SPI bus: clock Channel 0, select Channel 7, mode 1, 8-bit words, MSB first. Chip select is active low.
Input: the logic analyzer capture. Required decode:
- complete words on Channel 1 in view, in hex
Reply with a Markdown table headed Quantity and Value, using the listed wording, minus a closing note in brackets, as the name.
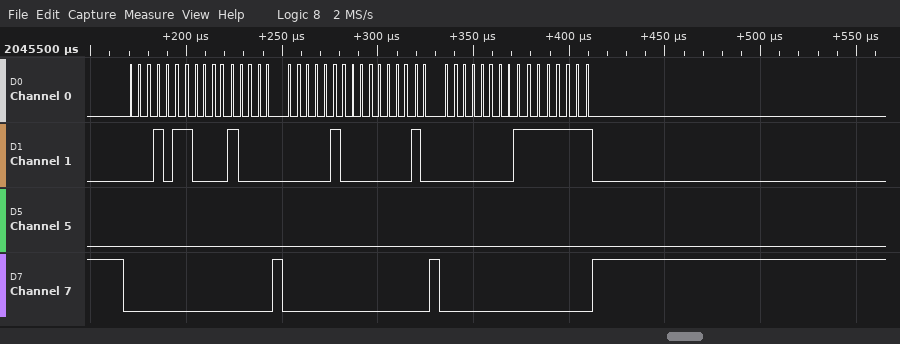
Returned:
| Quantity | Value |
|---|---|
| complete words on Channel 1 in view, in hex | 16, 10, 04, 02, 00, FF |
